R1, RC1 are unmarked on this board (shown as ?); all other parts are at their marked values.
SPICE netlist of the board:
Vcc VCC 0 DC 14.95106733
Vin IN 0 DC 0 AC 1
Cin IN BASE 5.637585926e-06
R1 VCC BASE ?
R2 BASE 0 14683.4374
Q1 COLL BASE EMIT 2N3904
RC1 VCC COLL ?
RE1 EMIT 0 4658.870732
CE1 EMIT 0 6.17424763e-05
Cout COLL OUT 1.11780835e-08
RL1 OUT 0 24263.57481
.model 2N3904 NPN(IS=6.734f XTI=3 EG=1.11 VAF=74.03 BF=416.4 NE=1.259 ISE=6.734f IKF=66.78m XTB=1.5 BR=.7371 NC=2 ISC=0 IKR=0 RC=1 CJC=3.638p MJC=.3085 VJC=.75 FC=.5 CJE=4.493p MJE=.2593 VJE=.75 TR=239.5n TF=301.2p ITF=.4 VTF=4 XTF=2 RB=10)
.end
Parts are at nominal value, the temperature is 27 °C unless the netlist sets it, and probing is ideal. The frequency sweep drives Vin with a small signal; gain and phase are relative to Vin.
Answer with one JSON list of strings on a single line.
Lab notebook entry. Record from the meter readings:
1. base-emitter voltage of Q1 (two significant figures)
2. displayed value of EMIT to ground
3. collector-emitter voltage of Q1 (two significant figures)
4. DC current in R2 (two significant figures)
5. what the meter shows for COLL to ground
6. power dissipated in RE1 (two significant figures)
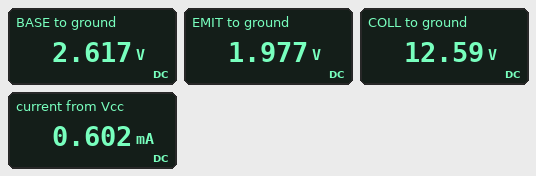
["640 mV", "1.977 V", "11 V", "180 µA", "12.59 V", "840 µW"]
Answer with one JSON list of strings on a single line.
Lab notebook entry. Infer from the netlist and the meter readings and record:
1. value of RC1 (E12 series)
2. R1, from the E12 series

["5.6 kΩ", "68 kΩ"]
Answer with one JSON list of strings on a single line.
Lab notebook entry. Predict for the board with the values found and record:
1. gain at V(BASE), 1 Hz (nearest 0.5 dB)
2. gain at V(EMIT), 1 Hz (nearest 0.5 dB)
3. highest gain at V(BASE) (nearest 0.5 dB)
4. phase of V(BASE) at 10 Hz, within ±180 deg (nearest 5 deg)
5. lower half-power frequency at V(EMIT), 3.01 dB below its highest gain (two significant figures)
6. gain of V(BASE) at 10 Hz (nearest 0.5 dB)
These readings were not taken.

["-8.5 dB", "-8.5 dB", "0 dB", "15 deg", "2.0 Hz", "-1.0 dB"]
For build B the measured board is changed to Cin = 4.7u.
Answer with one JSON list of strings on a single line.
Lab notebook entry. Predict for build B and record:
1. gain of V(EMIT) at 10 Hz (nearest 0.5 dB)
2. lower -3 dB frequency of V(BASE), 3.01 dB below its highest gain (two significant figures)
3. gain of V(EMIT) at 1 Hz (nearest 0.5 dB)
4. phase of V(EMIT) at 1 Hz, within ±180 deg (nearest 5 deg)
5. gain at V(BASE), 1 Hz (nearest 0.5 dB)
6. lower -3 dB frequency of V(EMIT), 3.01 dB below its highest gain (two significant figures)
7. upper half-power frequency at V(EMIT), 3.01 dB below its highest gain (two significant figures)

["-1.5 dB", "3.2 Hz", "-10.0 dB", "70 deg", "-9.5 dB", "2.4 Hz", "50 Hz"]
